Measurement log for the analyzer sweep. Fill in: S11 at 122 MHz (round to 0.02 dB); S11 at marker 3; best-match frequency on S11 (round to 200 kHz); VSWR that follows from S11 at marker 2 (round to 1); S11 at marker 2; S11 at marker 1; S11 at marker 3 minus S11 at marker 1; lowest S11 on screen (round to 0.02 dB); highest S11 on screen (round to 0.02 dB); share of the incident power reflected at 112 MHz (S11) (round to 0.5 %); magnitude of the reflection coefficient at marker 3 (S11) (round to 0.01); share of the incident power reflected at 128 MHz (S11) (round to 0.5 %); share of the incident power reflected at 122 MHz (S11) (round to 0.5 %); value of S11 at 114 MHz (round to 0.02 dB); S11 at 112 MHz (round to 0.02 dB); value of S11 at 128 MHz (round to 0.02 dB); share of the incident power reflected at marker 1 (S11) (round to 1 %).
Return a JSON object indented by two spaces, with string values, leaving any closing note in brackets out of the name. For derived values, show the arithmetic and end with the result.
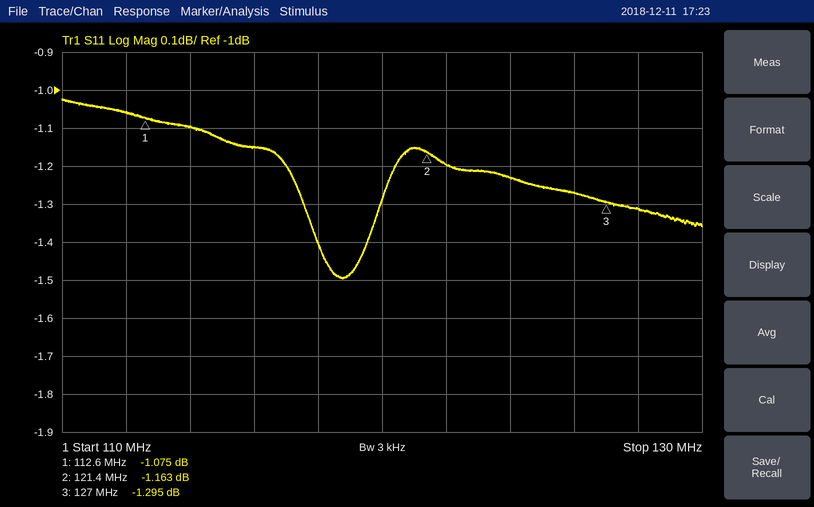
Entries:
{
  "S11 at 122 MHz": "-1.20 dB",
  "S11 at marker 3": "-1.295 dB",
  "best-match frequency on S11": "118.8 MHz",
  "VSWR that follows from S11 at marker 2": "(1 + 0.8747)/(1 − 0.8747) ≈ 15",
  "S11 at marker 2": "-1.163 dB",
  "S11 at marker 1": "-1.075 dB",
  "S11 at marker 3 minus S11 at marker 1": "-1.295 − (-1.075) = -0.220 dB",
  "lowest S11 on screen": "-1.50 dB",
  "highest S11 on screen": "-1.02 dB",
  "share of the incident power reflected at 112 MHz (S11)": "10^(-1.06/10) ≈ 78.3 %, so 78.5 % to the nearest 0.5 %",
  "magnitude of the reflection coefficient at marker 3 (S11)": "10^(-1.295/20) ≈ 0.86",
  "share of the incident power reflected at 128 MHz (S11)": "10^(-1.32/10) ≈ 73.8 %, so 74.0 % to the nearest 0.5 %",
  "share of the incident power reflected at 122 MHz (S11)": "10^(-1.2/10) ≈ 75.9 %, so 76.0 % to the nearest 0.5 %",
  "value of S11 at 114 MHz": "-1.10 dB",
  "S11 at 112 MHz": "-1.06 dB",
  "value of S11 at 128 MHz": "-1.32 dB",
  "share of the incident power reflected at marker 1 (S11)": "10^(-1.075/10) ≈ 78 %"
}
